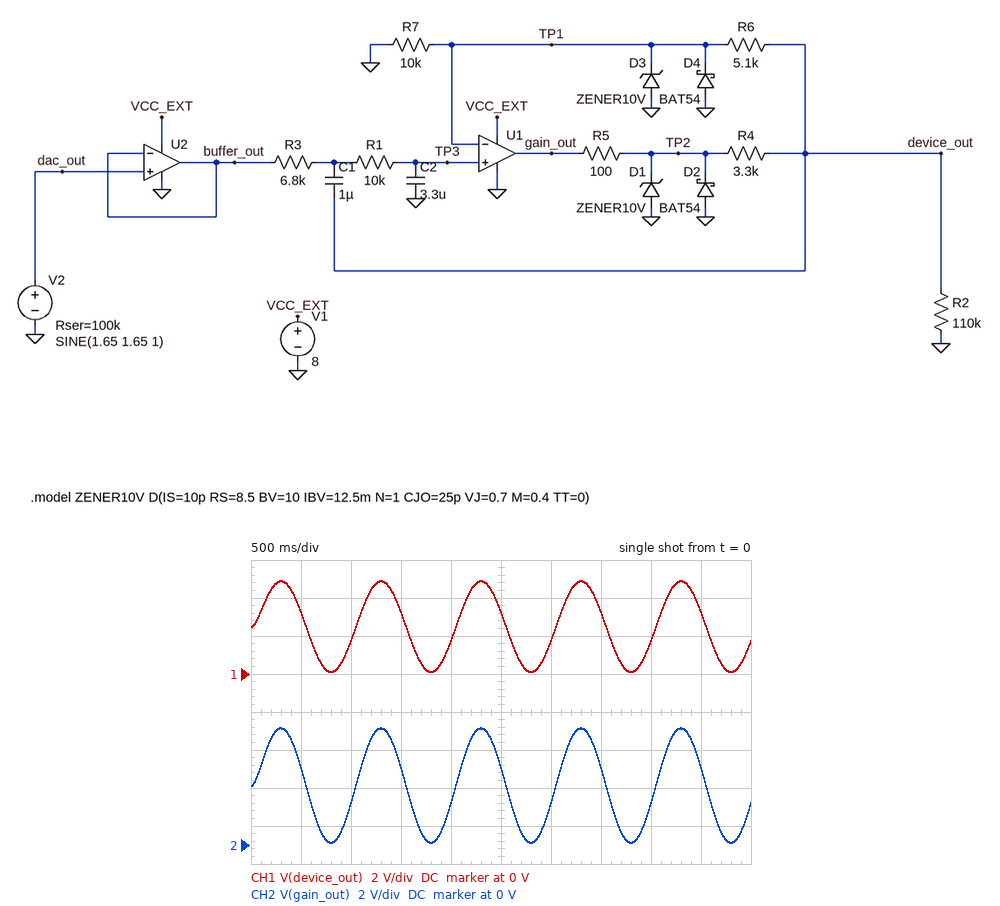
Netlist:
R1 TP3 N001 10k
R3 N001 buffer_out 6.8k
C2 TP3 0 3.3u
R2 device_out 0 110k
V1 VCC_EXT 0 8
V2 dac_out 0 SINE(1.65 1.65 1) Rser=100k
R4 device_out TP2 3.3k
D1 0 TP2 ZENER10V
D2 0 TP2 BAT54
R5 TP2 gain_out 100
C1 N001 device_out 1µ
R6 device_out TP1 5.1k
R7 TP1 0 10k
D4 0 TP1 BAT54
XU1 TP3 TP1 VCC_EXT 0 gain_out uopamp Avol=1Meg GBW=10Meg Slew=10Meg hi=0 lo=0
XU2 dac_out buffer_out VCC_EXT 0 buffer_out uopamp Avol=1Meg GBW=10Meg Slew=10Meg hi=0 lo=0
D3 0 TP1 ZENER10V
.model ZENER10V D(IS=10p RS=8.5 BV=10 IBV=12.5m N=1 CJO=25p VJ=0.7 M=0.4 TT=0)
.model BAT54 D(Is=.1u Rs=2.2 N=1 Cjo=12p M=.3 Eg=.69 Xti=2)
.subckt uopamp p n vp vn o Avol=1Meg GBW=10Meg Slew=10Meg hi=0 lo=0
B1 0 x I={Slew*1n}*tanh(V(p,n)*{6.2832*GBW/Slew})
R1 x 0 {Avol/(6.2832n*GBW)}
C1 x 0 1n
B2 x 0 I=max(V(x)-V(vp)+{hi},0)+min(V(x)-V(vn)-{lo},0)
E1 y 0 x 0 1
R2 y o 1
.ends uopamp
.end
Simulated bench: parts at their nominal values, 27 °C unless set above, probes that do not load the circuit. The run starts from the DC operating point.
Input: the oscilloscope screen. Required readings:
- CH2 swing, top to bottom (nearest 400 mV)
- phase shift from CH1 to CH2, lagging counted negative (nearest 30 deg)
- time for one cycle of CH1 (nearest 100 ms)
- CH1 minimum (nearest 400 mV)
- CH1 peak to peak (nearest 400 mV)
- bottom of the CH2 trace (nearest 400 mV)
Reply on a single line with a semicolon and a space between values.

6.0 V; 0 deg; 1.0 s; 0 V; 4.8 V; 0 V
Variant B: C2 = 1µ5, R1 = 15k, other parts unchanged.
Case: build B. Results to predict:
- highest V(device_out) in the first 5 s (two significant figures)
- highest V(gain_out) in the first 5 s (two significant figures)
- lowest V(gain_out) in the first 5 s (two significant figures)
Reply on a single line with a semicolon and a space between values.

5.0 V; 6.2 V; 29 mV
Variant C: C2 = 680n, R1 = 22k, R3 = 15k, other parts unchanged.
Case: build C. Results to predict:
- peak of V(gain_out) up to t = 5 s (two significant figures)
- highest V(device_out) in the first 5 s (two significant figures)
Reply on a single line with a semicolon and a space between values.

6.3 V; 5.0 V
